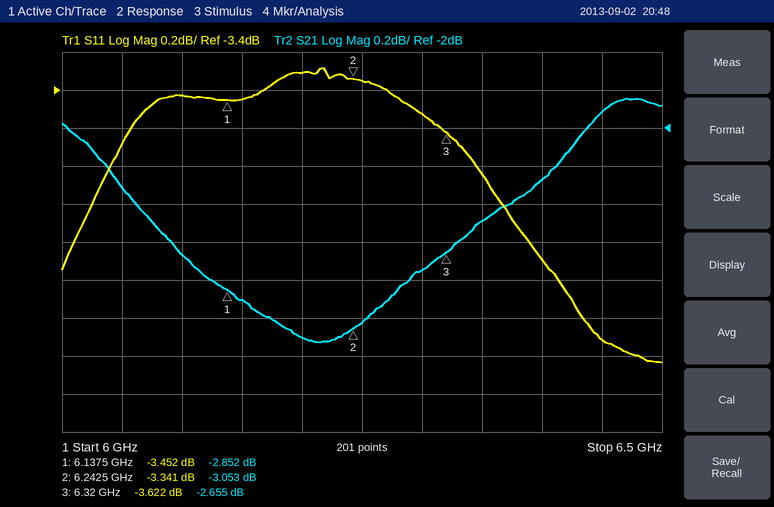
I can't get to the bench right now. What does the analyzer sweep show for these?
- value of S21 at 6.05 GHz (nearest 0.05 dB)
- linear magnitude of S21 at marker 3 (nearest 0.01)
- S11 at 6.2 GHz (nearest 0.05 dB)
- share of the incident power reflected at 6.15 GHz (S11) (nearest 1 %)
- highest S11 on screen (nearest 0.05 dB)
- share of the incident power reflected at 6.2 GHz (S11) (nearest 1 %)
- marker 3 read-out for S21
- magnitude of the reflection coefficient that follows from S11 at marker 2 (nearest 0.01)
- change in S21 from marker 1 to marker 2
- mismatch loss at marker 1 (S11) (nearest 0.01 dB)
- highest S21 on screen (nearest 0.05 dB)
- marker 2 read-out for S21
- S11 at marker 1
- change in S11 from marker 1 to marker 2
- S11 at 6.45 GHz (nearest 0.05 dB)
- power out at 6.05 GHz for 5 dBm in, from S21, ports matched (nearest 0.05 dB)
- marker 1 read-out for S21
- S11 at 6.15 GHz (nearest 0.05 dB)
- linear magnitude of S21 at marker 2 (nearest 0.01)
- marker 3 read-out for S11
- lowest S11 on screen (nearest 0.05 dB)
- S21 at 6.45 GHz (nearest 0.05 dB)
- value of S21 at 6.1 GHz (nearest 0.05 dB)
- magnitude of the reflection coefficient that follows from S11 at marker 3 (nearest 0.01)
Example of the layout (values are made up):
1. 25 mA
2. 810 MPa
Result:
1. -2.30 dB
2. 0.74
3. -3.30 dB
4. 45 %
5. -3.30 dB
6. 47 %
7. -2.655 dB
8. 0.68
9. -0.201 dB
10. 2.61 dB
11. -1.85 dB
12. -3.053 dB
13. -3.452 dB
14. 0.111 dB
15. -4.70 dB
16. 2.70 dBm
17. -2.852 dB
18. -3.45 dB
19. 0.70
20. -3.622 dB
21. -4.85 dB
22. -1.90 dB
23. -2.65 dB
24. 0.66
